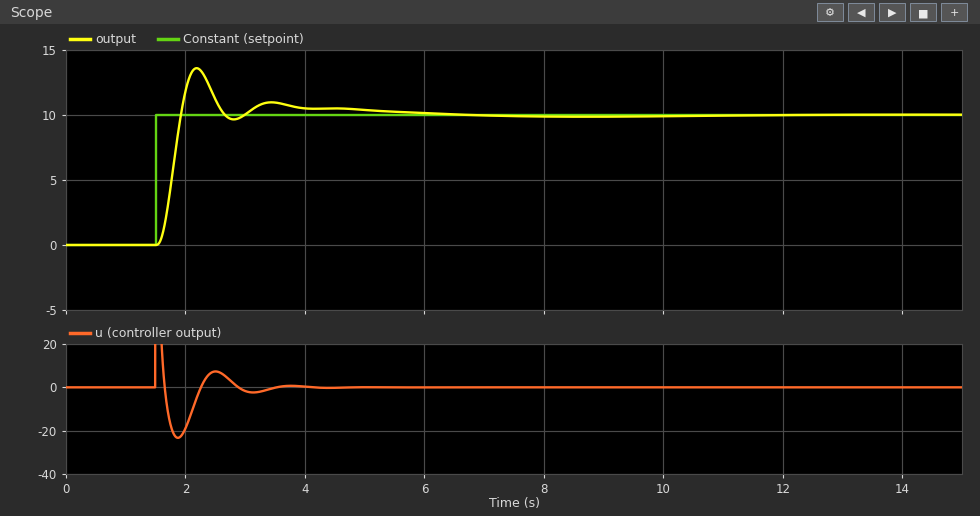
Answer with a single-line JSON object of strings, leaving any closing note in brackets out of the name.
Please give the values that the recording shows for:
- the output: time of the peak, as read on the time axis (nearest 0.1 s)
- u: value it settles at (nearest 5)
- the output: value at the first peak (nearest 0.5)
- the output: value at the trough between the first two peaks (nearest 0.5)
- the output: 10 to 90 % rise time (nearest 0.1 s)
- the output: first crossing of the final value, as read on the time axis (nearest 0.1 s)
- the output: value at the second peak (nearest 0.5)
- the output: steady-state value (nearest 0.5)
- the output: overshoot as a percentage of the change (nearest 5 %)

{"the output: time of the peak, as read on the time axis": "2.2 s", "u: value it settles at": "0", "the output: value at the first peak": "13.5", "the output: value at the trough between the first two peaks": "9.5", "the output: 10 to 90 % rise time": "0.3 s", "the output: first crossing of the final value, as read on the time axis": "1.9 s", "the output: value at the second peak": "11.0", "the output: steady-state value": "10.0", "the output: overshoot as a percentage of the change": "35 %"}
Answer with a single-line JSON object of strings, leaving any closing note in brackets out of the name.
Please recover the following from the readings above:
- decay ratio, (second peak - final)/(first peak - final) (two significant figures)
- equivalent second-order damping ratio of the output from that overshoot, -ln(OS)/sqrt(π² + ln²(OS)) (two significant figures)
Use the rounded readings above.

{"decay ratio, (second peak - final)/(first peak - final)": "0.29", "equivalent second-order damping ratio of the output from that overshoot, -ln(OS)/sqrt(π² + ln²(OS))": "0.32"}
